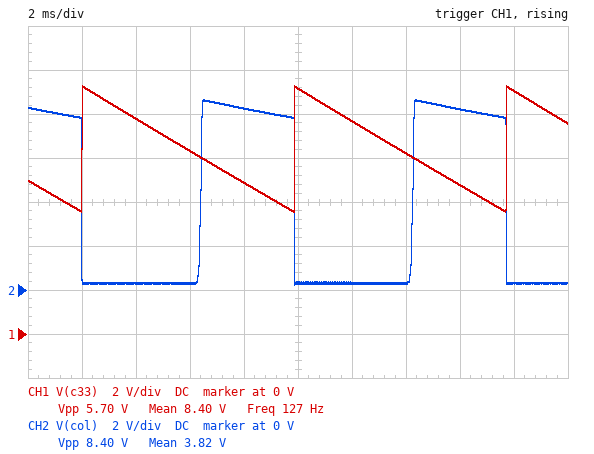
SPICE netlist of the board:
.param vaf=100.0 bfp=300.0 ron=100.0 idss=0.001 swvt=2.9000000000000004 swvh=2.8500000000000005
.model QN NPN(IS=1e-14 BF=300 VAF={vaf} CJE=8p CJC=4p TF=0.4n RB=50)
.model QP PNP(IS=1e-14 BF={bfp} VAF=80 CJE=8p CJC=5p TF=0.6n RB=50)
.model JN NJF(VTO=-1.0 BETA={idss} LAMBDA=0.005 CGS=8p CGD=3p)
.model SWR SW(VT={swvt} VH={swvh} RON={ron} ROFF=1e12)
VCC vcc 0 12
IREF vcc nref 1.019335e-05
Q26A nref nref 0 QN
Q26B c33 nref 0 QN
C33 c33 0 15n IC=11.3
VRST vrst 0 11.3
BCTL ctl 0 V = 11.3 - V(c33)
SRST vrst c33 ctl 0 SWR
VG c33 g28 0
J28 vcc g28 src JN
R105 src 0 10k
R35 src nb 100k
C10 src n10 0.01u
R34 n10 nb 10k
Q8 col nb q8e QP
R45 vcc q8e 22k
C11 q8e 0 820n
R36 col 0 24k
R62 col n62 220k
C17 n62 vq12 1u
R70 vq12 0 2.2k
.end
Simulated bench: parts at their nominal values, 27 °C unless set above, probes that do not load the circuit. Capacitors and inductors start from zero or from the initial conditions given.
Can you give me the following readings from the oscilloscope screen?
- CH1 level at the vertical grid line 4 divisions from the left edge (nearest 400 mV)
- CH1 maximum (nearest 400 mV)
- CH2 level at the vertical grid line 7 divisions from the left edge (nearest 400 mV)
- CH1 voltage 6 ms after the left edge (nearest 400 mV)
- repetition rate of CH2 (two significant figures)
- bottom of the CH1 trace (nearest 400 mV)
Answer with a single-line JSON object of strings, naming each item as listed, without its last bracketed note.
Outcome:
{"CH1 level at the vertical grid line 4 divisions from the left edge": "6.8 V", "CH1 maximum": "11.2 V", "CH2 level at the vertical grid line 7 divisions from the left edge": "400 mV", "CH1 voltage 6 ms after the left edge": "8.4 V", "repetition rate of CH2": "130 Hz", "bottom of the CH1 trace": "5.6 V"}
